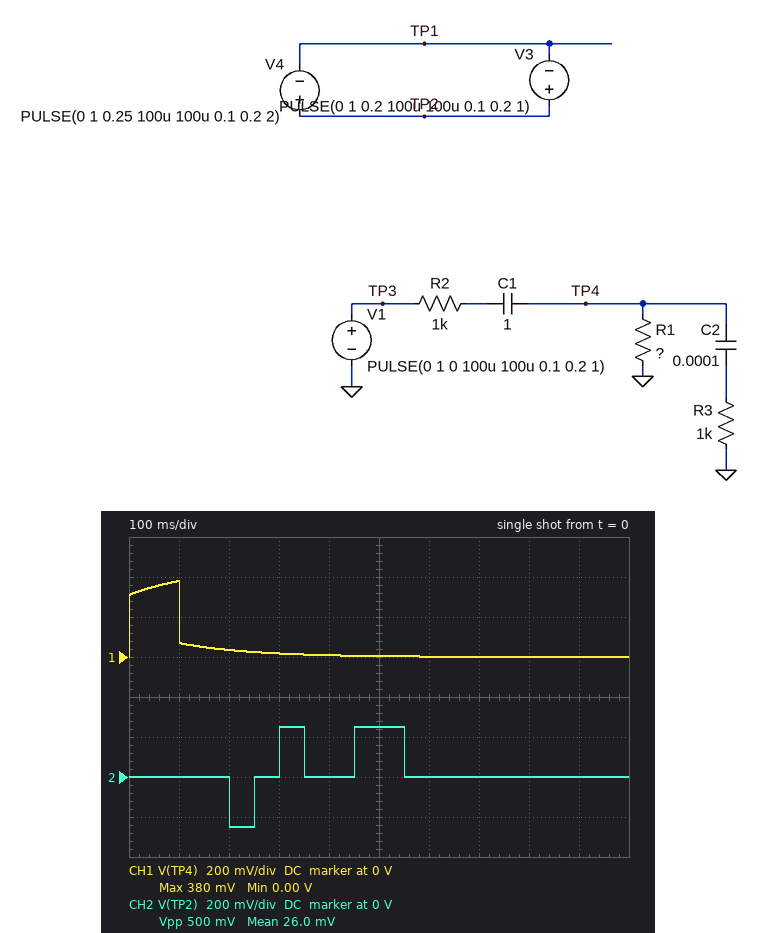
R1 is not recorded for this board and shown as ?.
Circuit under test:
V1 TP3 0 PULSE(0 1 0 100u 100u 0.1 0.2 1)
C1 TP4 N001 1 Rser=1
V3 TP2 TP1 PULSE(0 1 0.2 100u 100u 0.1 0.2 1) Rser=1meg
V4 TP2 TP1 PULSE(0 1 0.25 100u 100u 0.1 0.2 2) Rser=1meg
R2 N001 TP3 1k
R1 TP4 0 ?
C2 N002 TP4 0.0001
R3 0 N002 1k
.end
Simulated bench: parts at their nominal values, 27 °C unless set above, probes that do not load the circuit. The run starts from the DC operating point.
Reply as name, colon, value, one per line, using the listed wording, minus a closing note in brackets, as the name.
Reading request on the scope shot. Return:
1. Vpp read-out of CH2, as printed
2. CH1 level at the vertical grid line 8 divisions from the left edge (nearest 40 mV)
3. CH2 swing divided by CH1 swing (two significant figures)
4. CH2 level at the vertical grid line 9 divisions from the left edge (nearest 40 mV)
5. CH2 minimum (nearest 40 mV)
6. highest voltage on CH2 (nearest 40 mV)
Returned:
Vpp read-out of CH2, as printed: 500 mV
CH1 level at the vertical grid line 8 divisions from the left edge: 0 V
CH2 swing divided by CH1 swing: 1.3
CH2 level at the vertical grid line 9 divisions from the left edge: 0 V
CH2 minimum: -240 mV
highest voltage on CH2: 240 mV
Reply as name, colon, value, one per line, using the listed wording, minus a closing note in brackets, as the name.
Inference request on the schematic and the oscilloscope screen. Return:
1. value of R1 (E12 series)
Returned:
value of R1: 820 Ω
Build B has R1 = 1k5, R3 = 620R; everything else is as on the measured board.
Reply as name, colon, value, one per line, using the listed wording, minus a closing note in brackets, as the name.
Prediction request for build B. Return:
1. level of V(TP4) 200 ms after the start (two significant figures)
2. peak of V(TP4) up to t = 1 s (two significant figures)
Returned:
level of V(TP4) 200 ms after the start: 73 mV
peak of V(TP4) up to t = 1 s: 470 mV
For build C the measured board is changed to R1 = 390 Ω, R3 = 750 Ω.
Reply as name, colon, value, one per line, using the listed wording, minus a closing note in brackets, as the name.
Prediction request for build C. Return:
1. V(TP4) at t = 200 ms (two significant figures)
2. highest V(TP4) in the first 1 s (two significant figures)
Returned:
V(TP4) at t = 200 ms: 18 mV
highest V(TP4) in the first 1 s: 250 mV
